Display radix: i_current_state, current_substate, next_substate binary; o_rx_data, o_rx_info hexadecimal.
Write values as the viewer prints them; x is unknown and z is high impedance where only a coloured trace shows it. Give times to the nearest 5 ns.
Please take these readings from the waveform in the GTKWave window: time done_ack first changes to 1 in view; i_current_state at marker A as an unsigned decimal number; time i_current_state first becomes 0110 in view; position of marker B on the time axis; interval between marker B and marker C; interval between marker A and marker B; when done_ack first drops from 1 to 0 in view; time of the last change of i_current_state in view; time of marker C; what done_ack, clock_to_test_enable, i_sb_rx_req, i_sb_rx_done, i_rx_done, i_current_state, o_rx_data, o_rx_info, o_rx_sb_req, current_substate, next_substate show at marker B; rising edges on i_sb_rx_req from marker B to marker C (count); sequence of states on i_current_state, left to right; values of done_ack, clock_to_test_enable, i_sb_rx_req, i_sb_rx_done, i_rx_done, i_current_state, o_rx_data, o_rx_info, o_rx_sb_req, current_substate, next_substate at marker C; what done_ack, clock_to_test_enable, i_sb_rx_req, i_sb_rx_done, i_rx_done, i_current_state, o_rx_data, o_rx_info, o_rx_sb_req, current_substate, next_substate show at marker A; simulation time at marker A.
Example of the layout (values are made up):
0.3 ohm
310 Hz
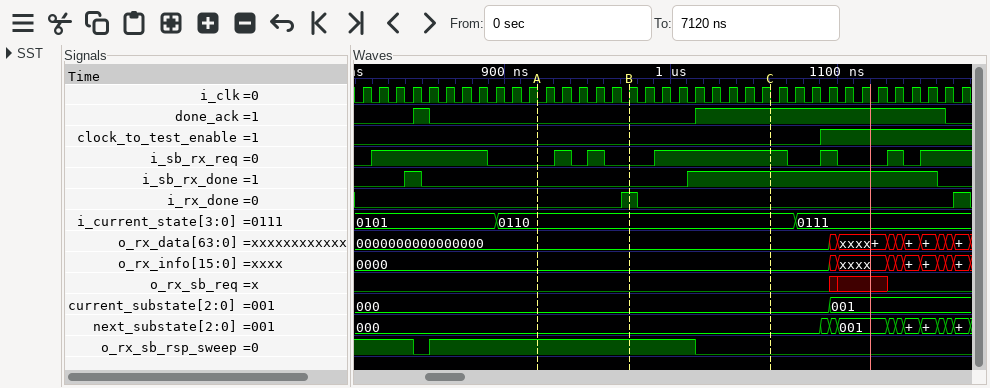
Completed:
845 ns
6
895 ns
975 ns
85 ns
55 ns
855 ns
1075 ns
1060 ns
done_ack=0, clock_to_test_enable=0, i_sb_rx_req=0, i_sb_rx_done=0, i_rx_done=1, i_current_state=0110, o_rx_data=0000000000000000, o_rx_info=0000, o_rx_sb_req=0, current_substate=000, next_substate=000
1
0101, 0110, 0111
done_ack=1, clock_to_test_enable=0, i_sb_rx_req=1, i_sb_rx_done=1, i_rx_done=0, i_current_state=0110, o_rx_data=0000000000000000, o_rx_info=0000, o_rx_sb_req=0, current_substate=000, next_substate=000
done_ack=0, clock_to_test_enable=0, i_sb_rx_req=0, i_sb_rx_done=0, i_rx_done=0, i_current_state=0110, o_rx_data=0000000000000000, o_rx_info=0000, o_rx_sb_req=0, current_substate=000, next_substate=000
920 ns
